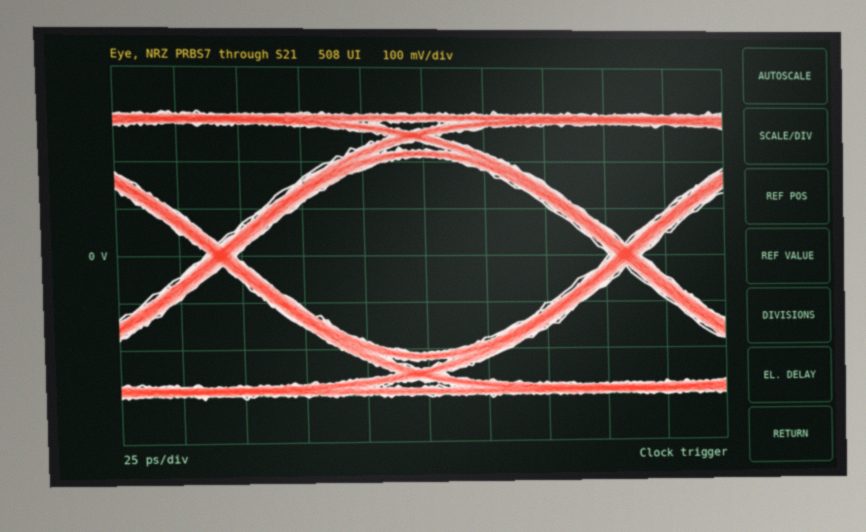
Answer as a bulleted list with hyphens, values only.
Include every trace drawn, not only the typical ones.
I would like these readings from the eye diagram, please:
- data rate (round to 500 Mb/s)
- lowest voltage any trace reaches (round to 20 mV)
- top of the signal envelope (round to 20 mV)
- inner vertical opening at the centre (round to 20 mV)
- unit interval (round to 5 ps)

- 6.0 Gb/s
- -300 mV
- 300 mV
- 420 mV
- 165 ps
